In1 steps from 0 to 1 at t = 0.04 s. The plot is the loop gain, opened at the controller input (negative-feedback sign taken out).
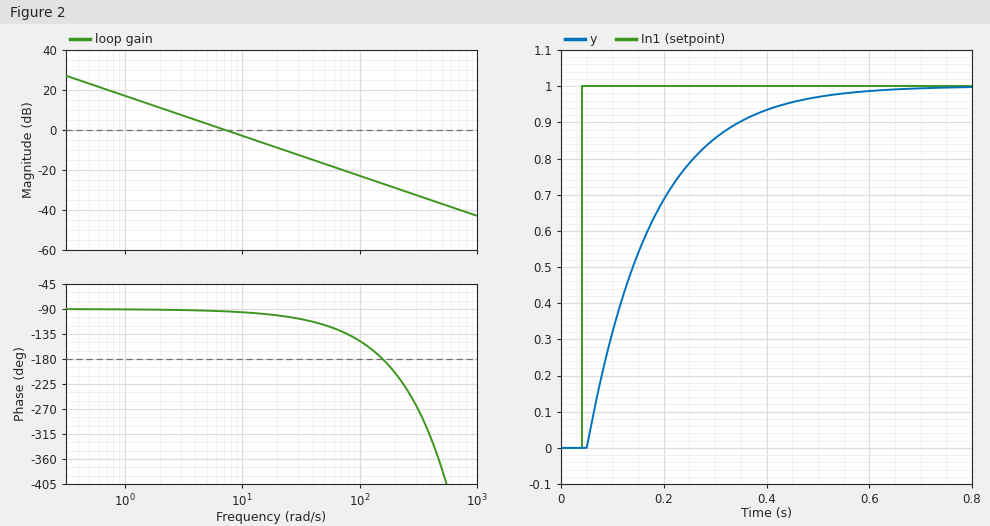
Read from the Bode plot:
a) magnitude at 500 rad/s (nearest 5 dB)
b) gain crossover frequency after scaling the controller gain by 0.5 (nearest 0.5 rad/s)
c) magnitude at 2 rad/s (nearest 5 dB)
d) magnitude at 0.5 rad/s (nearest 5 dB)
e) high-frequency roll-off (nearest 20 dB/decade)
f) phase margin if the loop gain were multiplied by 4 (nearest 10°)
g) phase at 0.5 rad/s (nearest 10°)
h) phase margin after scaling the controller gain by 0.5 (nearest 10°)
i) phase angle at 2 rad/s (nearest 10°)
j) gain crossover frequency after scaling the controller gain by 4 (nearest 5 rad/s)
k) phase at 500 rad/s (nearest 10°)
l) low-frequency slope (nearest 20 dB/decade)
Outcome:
-35 dB
3.5 rad/s
10 dB
25 dB
-20 dB/decade
70°
-90°
90°
-90°
30 rad/s
-380°
-20 dB/decade
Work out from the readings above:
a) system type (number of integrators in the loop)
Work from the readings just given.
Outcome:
1
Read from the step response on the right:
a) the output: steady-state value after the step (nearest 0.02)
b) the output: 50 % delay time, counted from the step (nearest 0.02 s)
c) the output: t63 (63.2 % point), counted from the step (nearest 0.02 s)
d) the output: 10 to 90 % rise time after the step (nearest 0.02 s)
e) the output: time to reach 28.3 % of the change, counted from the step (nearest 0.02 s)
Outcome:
1.00
0.10 s
0.14 s
0.28 s
0.06 s
